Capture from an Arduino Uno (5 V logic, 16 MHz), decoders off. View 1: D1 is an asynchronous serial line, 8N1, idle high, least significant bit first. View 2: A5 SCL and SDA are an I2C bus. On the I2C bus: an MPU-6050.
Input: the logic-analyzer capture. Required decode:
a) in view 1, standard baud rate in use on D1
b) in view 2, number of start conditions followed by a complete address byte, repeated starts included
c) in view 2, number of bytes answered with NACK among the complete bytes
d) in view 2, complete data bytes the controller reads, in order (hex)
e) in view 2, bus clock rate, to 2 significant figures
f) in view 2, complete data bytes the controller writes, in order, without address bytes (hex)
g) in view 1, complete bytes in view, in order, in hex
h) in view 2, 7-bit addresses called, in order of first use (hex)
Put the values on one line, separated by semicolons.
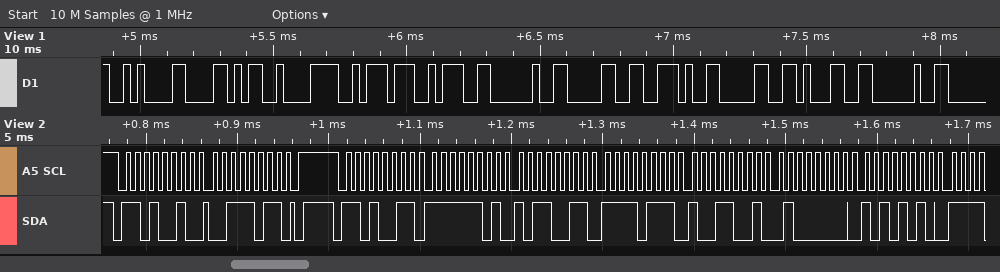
38400 baud; 2; 0; FD B3 F7 99 40 AA; 100 kHz; 3B; 0x0A 0x58 0xC2 0xBA 0x3A 0x20 0x30 0x2E 0x30 0x31 0x20; 0x69
